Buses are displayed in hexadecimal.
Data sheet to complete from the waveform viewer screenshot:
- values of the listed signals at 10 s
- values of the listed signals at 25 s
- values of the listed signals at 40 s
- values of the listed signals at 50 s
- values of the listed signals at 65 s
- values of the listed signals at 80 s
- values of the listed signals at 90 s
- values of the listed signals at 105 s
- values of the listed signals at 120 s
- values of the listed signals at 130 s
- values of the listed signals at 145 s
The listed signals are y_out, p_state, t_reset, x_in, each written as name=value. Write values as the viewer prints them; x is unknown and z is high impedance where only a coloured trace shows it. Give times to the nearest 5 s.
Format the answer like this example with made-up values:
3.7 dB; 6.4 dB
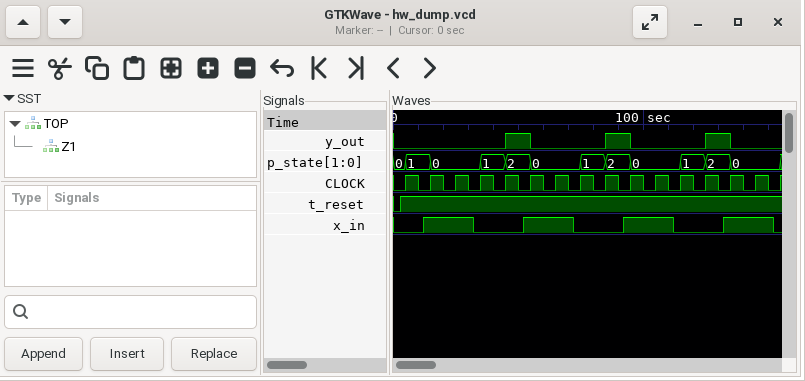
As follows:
y_out=0, p_state=1, t_reset=1, x_in=0; y_out=0, p_state=0, t_reset=1, x_in=1; y_out=0, p_state=1, t_reset=1, x_in=0; y_out=1, p_state=2, t_reset=1, x_in=0; y_out=0, p_state=0, t_reset=1, x_in=1; y_out=0, p_state=1, t_reset=1, x_in=0; y_out=1, p_state=2, t_reset=1, x_in=0; y_out=0, p_state=0, t_reset=1, x_in=1; y_out=0, p_state=1, t_reset=1, x_in=0; y_out=1, p_state=2, t_reset=1, x_in=0; y_out=0, p_state=0, t_reset=1, x_in=1
